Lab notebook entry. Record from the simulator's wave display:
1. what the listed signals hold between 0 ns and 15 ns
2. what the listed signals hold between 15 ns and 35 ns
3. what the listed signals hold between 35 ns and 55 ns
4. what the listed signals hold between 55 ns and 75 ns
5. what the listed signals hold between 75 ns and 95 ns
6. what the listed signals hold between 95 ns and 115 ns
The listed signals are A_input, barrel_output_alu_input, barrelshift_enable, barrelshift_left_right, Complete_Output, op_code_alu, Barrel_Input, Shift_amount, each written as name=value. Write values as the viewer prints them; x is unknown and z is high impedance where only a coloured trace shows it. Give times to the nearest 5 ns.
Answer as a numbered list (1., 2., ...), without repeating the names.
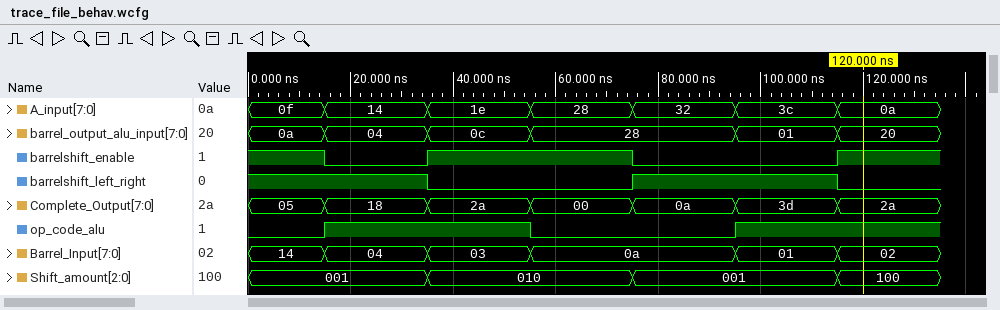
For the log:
1. A_input=0f, barrel_output_alu_input=0a, barrelshift_enable=1, barrelshift_left_right=1, Complete_Output=05, op_code_alu=0, Barrel_Input=14, Shift_amount=001
2. A_input=14, barrel_output_alu_input=04, barrelshift_enable=0, barrelshift_left_right=1, Complete_Output=18, op_code_alu=1, Barrel_Input=04, Shift_amount=001
3. A_input=1e, barrel_output_alu_input=0c, barrelshift_enable=1, barrelshift_left_right=0, Complete_Output=2a, op_code_alu=1, Barrel_Input=03, Shift_amount=010
4. A_input=28, barrel_output_alu_input=28, barrelshift_enable=1, barrelshift_left_right=0, Complete_Output=00, op_code_alu=0, Barrel_Input=0a, Shift_amount=010
5. A_input=32, barrel_output_alu_input=28, barrelshift_enable=0, barrelshift_left_right=1, Complete_Output=0a, op_code_alu=0, Barrel_Input=0a, Shift_amount=001
6. A_input=3c, barrel_output_alu_input=01, barrelshift_enable=0, barrelshift_left_right=1, Complete_Output=3d, op_code_alu=1, Barrel_Input=01, Shift_amount=001
